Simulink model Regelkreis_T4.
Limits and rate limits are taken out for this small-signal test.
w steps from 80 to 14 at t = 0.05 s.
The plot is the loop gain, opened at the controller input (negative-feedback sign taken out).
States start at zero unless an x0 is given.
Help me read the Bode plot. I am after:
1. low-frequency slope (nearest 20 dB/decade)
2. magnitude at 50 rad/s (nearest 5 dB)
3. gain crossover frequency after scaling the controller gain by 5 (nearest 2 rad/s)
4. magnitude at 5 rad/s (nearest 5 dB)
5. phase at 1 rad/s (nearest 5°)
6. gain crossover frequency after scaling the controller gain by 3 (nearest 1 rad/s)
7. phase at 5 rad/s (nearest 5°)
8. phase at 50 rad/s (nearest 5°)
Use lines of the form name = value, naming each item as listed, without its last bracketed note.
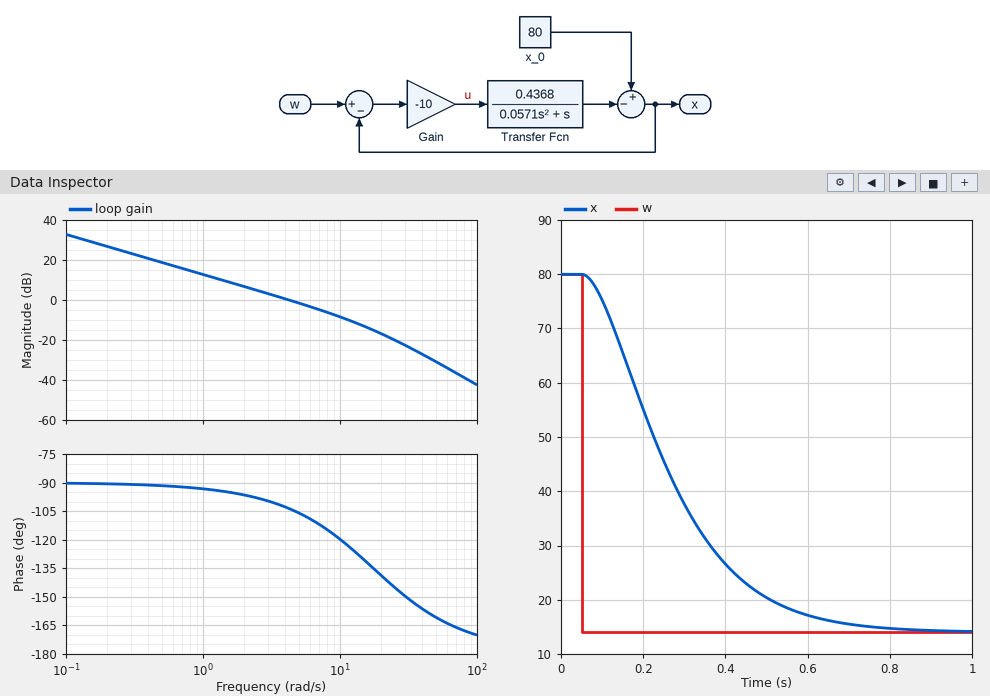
low-frequency slope = -20 dB/decade
magnitude at 50 rad/s = -30 dB
gain crossover frequency after scaling the controller gain by 5 = 16 rad/s
magnitude at 5 rad/s = 0 dB
phase at 1 rad/s = -95°
gain crossover frequency after scaling the controller gain by 3 = 11 rad/s
phase at 5 rad/s = -105°
phase at 50 rad/s = -160°
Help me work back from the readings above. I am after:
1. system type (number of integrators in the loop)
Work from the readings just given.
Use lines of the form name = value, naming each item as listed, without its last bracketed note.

system type = 1
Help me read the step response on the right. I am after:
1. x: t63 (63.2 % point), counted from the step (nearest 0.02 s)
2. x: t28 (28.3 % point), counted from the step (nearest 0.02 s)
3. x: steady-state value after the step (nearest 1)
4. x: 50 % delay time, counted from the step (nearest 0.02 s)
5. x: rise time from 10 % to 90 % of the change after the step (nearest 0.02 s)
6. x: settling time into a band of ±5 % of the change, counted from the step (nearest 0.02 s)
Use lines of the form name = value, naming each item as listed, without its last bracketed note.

x: t63 (63.2 % point), counted from the step = 0.24 s
x: t28 (28.3 % point), counted from the step = 0.12 s
x: steady-state value after the step = 14
x: 50 % delay time, counted from the step = 0.20 s
x: rise time from 10 % to 90 % of the change after the step = 0.38 s
x: settling time into a band of ±5 % of the change, counted from the step = 0.54 s
